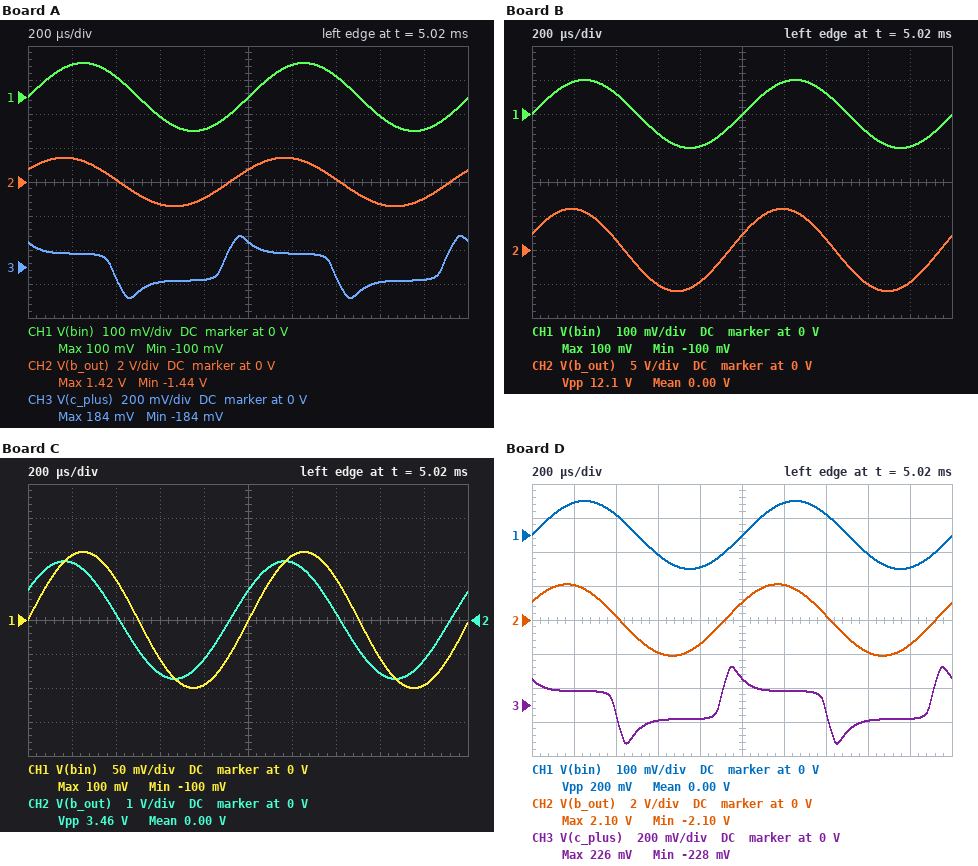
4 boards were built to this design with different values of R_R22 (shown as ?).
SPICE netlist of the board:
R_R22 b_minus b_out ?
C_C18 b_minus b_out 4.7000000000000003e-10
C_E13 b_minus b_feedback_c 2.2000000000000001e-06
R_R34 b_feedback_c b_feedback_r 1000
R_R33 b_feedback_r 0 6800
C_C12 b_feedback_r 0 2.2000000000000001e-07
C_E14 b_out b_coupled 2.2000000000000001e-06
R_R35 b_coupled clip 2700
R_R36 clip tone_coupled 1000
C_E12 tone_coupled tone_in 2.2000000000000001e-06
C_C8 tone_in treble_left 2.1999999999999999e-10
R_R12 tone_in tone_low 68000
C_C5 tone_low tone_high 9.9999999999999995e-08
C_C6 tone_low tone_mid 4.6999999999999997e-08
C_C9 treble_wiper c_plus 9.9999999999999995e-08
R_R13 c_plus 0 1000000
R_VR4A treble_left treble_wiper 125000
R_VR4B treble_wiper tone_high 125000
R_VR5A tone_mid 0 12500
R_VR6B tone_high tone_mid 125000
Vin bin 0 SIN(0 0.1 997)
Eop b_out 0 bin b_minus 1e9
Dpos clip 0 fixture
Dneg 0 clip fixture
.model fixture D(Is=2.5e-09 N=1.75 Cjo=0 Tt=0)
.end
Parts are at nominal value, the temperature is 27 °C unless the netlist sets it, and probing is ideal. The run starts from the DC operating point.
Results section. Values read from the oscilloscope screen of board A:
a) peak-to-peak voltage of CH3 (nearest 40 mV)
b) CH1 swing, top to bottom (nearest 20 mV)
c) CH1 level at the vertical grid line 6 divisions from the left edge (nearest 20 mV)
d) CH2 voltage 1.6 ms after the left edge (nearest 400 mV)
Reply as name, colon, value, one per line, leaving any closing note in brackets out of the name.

peak-to-peak voltage of CH3: 360 mV
CH1 swing, top to bottom: 200 mV
CH1 level at the vertical grid line 6 divisions from the left edge: 100 mV
CH2 voltage 1.6 ms after the left edge: -1.2 V
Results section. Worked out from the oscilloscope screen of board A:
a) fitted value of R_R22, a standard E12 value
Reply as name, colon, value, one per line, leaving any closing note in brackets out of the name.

fitted value of R_R22, a standard E12 value: 18 kΩ
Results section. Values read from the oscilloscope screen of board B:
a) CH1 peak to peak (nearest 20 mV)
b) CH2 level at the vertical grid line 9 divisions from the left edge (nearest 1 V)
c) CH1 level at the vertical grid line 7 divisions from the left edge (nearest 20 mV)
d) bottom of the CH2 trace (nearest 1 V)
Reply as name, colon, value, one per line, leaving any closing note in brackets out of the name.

CH1 peak to peak: 200 mV
CH2 level at the vertical grid line 9 divisions from the left edge: -5 V
CH1 level at the vertical grid line 7 divisions from the left edge: 60 mV
bottom of the CH2 trace: -6 V
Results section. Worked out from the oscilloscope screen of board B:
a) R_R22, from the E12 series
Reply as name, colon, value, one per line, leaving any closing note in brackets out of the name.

R_R22, from the E12 series: 82 kΩ
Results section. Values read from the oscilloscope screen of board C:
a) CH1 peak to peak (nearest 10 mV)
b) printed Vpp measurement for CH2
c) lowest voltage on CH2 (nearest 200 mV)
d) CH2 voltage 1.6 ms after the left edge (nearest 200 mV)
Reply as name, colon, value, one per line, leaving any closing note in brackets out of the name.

CH1 peak to peak: 200 mV
printed Vpp measurement for CH2: 3.46 V
lowest voltage on CH2: -1.8 V
CH2 voltage 1.6 ms after the left edge: -1.6 V
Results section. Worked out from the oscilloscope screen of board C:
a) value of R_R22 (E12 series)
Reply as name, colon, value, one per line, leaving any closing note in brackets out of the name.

value of R_R22: 22 kΩ
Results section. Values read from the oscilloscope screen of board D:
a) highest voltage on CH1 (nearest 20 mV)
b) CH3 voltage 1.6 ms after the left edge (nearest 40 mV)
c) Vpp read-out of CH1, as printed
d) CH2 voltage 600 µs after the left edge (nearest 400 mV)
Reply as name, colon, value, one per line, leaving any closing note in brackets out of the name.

highest voltage on CH1: 100 mV
CH3 voltage 1.6 ms after the left edge: -80 mV
Vpp read-out of CH1, as printed: 200 mV
CH2 voltage 600 µs after the left edge: -2.0 V
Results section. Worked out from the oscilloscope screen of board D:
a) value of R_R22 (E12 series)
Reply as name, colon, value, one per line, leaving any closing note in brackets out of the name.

value of R_R22: 27 kΩ
